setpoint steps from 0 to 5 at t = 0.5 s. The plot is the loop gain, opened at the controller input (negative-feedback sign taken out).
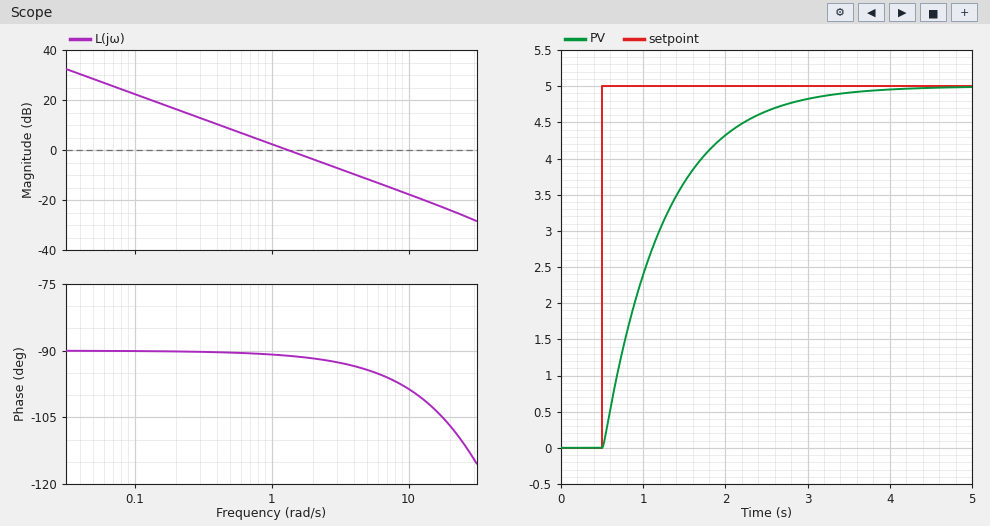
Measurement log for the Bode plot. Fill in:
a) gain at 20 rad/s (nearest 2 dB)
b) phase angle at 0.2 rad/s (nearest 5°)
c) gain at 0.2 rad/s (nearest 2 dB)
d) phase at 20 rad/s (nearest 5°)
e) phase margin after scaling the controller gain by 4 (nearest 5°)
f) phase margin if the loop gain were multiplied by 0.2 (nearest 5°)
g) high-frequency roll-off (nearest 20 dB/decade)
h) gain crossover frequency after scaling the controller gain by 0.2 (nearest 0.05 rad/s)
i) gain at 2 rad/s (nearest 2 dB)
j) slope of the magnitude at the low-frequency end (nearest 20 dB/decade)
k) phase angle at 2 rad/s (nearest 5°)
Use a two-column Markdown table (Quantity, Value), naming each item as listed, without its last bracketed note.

| Quantity | Value |
|---|---|
| gain at 20 rad/s | -24 dB |
| phase angle at 0.2 rad/s | -90° |
| gain at 0.2 rad/s | 16 dB |
| phase at 20 rad/s | -105° |
| phase margin after scaling the controller gain by 4 | 85° |
| phase margin if the loop gain were multiplied by 0.2 | 90° |
| high-frequency roll-off | -20 dB/decade |
| gain crossover frequency after scaling the controller gain by 0.2 | 0.25 rad/s |
| gain at 2 rad/s | -4 dB |
| slope of the magnitude at the low-frequency end | -20 dB/decade |
| phase angle at 2 rad/s | -90° |
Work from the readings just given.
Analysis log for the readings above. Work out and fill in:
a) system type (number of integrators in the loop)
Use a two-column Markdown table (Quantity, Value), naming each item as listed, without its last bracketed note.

| Quantity | Value |
|---|---|
| system type | 1 |
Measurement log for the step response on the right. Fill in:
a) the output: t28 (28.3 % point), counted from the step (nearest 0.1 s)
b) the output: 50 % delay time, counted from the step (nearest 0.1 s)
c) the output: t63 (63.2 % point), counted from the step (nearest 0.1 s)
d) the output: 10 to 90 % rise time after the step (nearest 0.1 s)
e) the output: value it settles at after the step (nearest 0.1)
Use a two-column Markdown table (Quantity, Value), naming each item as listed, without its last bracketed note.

| Quantity | Value |
|---|---|
| the output: t28 (28.3 % point), counted from the step | 0.3 s |
| the output: 50 % delay time, counted from the step | 0.5 s |
| the output: t63 (63.2 % point), counted from the step | 0.8 s |
| the output: 10 to 90 % rise time after the step | 1.6 s |
| the output: value it settles at after the step | 5.0 |
